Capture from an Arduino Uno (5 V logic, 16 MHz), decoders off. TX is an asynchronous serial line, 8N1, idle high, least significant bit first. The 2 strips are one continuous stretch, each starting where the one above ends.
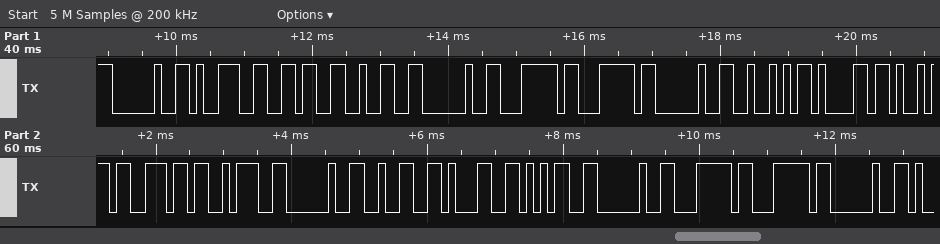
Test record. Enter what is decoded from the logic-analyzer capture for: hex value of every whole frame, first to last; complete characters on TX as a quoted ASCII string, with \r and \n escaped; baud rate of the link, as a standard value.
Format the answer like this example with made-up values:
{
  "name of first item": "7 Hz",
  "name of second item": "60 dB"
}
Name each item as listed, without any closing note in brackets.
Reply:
{
  "hex value of every whole frame, first to last": "20 39 36 32 20 7C 7C 20 52 61 69 6E 3A 20 32 31 35 20 7C 7C 20",
  "complete characters on TX as a quoted ASCII string, with \\r and \\n escaped": "\" 962 || Rain: 215 || \"",
  "baud rate of the link, as a standard value": "9600 baud"
}
